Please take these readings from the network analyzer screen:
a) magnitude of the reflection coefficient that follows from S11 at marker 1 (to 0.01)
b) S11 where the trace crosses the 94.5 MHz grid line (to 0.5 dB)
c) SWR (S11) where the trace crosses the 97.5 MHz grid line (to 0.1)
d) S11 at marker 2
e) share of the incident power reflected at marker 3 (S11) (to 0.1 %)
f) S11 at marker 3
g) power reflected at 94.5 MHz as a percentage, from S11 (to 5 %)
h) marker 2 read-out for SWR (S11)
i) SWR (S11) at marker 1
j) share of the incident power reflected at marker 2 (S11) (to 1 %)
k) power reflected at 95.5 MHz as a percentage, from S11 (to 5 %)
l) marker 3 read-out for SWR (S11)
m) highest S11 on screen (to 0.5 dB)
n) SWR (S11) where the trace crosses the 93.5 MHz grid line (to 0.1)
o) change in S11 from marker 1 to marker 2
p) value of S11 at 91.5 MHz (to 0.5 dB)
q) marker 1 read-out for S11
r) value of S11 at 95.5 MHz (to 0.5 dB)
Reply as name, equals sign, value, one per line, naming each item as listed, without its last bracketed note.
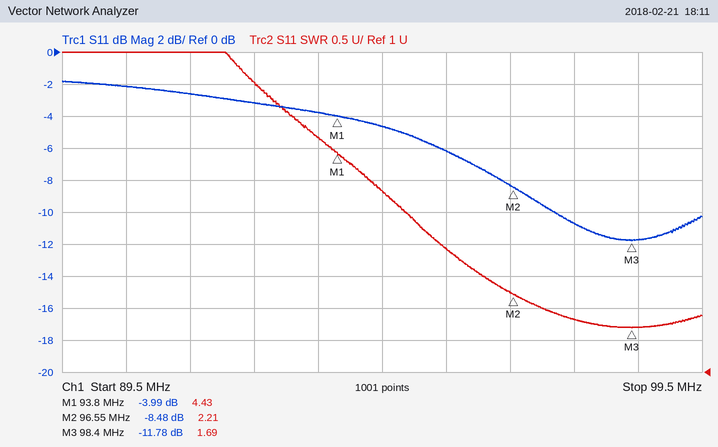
magnitude of the reflection coefficient that follows from S11 at marker 1 = 0.63
S11 where the trace crosses the 94.5 MHz grid line = -4.5 dB
SWR (S11) where the trace crosses the 97.5 MHz grid line = 1.8
S11 at marker 2 = -8.48 dB
share of the incident power reflected at marker 3 (S11) = 6.6 %
S11 at marker 3 = -11.78 dB
power reflected at 94.5 MHz as a percentage, from S11 = 35 %
marker 2 read-out for SWR = 2.21
SWR (S11) at marker 1 = 4.43
share of the incident power reflected at marker 2 (S11) = 14 %
power reflected at 95.5 MHz as a percentage, from S11 = 25 %
marker 3 read-out for SWR = 1.69
highest S11 on screen = -2.0 dB
SWR (S11) where the trace crosses the 93.5 MHz grid line = 4.7
change in S11 from marker 1 to marker 2 = -4.49 dB
value of S11 at 91.5 MHz = -2.5 dB
marker 1 read-out for S11 = -3.99 dB
value of S11 at 95.5 MHz = -6.0 dB
